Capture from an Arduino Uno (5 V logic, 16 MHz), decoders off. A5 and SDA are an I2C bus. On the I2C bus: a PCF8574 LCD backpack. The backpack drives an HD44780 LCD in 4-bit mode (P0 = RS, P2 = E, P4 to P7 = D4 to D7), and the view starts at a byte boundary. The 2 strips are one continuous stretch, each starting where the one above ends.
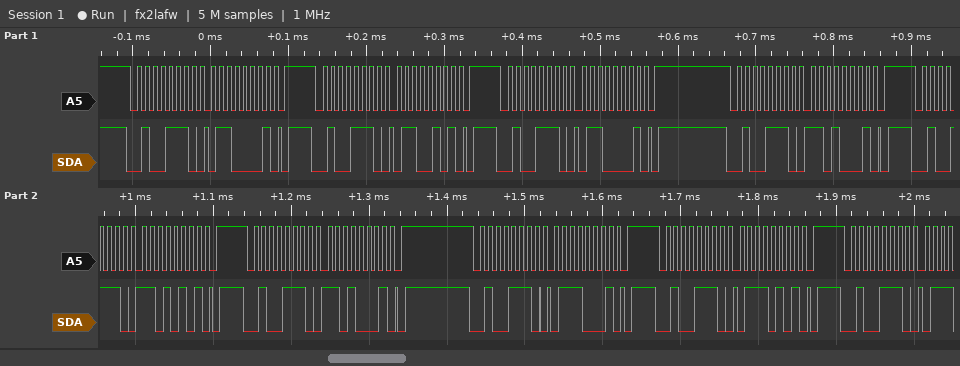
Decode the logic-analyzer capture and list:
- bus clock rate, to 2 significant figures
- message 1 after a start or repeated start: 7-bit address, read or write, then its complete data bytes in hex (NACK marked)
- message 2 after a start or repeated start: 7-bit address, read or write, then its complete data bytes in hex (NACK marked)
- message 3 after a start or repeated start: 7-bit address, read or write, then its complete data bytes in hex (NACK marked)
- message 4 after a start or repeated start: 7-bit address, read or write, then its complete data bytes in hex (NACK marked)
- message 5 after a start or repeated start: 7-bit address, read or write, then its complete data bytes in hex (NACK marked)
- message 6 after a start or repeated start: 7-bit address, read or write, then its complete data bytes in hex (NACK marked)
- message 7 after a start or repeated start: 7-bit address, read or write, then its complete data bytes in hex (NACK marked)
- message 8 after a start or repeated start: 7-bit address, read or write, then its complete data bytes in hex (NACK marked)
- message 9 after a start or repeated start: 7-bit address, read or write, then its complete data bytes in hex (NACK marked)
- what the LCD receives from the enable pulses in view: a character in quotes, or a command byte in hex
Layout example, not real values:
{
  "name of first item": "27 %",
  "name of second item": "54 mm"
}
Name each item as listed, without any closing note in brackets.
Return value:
{
  "bus clock rate, to 2 significant figures": "100 kHz",
  "message 1 after a start or repeated start: 7-bit address, read or write, then its complete data bytes in hex": "0x27 write: 61",
  "message 2 after a start or repeated start: 7-bit address, read or write, then its complete data bytes in hex": "0x27 write: 65",
  "message 3 after a start or repeated start: 7-bit address, read or write, then its complete data bytes in hex": "0x27 write: 61",
  "message 4 after a start or repeated start: 7-bit address, read or write, then its complete data bytes in hex": "0x27 write: D1",
  "message 5 after a start or repeated start: 7-bit address, read or write, then its complete data bytes in hex": "0x27 write: D5",
  "message 6 after a start or repeated start: 7-bit address, read or write, then its complete data bytes in hex": "0x27 write: D1",
  "message 7 after a start or repeated start: 7-bit address, read or write, then its complete data bytes in hex": "0x27 write: 71",
  "message 8 after a start or repeated start: 7-bit address, read or write, then its complete data bytes in hex": "0x27 write: 75",
  "message 9 after a start or repeated start: 7-bit address, read or write, then its complete data bytes in hex": "0x27 write",
  "what the LCD receives from the enable pulses in view: a character in quotes, or a command byte in hex": "'m'"
}
